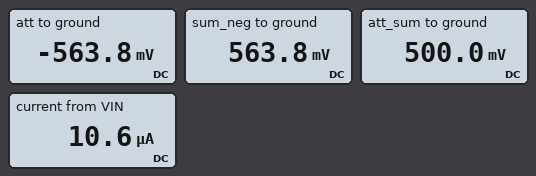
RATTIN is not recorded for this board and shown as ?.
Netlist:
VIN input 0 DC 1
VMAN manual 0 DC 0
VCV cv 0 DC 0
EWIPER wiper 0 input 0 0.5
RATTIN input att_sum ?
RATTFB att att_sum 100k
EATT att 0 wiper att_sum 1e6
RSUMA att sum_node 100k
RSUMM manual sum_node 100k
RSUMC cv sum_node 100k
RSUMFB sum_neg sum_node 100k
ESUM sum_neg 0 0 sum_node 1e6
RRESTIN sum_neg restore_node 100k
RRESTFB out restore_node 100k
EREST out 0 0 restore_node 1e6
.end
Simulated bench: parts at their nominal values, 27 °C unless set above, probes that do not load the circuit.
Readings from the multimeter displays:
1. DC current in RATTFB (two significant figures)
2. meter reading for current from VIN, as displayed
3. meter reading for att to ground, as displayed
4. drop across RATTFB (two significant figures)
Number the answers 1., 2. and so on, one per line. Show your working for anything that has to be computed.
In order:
1. (500 mV - (-563.8 mV)) / 100 kΩ = 11 µA
2. 10.6 µA
3. -563.8 mV
4. 500 mV - (-563.8 mV) = 1.1 V
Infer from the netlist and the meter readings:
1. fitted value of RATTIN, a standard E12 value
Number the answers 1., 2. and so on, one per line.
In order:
1. 47 kΩ
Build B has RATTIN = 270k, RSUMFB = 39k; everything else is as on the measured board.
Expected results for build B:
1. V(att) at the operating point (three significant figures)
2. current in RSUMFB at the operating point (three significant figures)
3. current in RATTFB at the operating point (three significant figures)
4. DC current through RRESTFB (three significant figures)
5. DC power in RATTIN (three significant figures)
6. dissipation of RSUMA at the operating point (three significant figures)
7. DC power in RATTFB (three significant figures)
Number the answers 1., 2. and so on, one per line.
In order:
1. 315 mV
2. 3.15 µA
3. 1.85 µA
4. 1.23 µA
5. 926 nW
6. 991 nW
7. 343 nW
